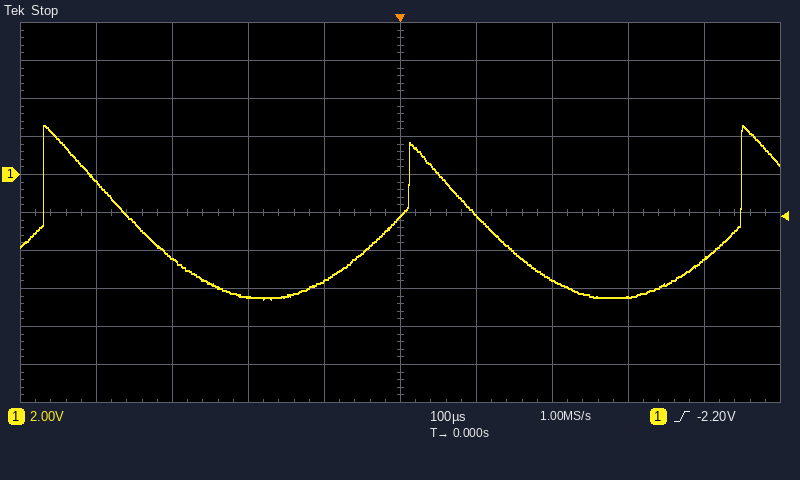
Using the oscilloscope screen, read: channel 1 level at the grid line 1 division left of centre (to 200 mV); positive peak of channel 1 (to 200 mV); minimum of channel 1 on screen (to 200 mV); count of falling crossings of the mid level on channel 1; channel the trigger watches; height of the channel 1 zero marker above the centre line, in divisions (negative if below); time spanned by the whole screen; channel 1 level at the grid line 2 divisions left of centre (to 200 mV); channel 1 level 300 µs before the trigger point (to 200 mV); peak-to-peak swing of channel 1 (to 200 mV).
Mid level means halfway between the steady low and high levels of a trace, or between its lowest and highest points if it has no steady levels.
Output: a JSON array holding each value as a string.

["-5.6 V", "2.6 V", "-6.6 V", "2", "channel 1", "+1.0 div", "1 ms", "-6.4 V", "-4.4 V", "9.2 V"]
